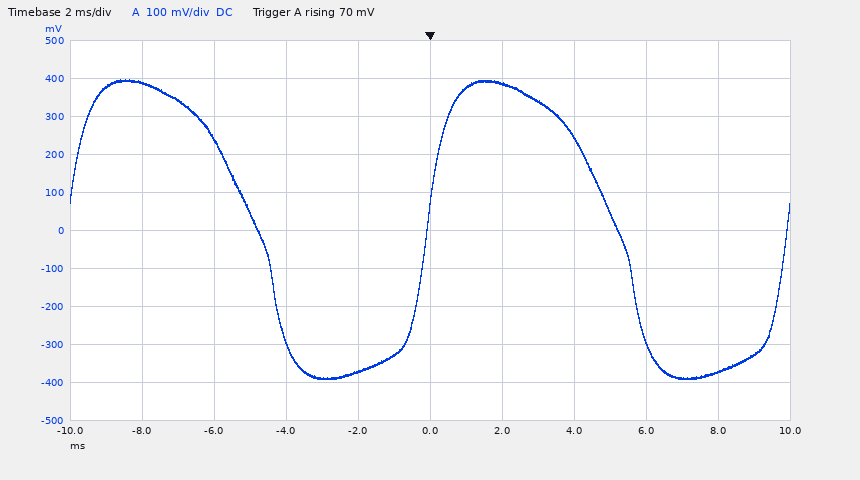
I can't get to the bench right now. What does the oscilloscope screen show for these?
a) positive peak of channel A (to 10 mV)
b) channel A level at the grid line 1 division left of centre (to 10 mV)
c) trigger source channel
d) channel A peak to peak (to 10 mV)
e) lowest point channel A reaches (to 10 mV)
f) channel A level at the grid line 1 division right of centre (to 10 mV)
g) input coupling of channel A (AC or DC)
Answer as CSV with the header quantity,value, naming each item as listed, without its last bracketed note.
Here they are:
quantity,value
positive peak of channel A,400 mV
channel A level at the grid line 1 division left of centre,-370 mV
trigger source channel,channel A
channel A peak to peak,790 mV
lowest point channel A reaches,-390 mV
channel A level at the grid line 1 division right of centre,390 mV
input coupling of channel A,DC
